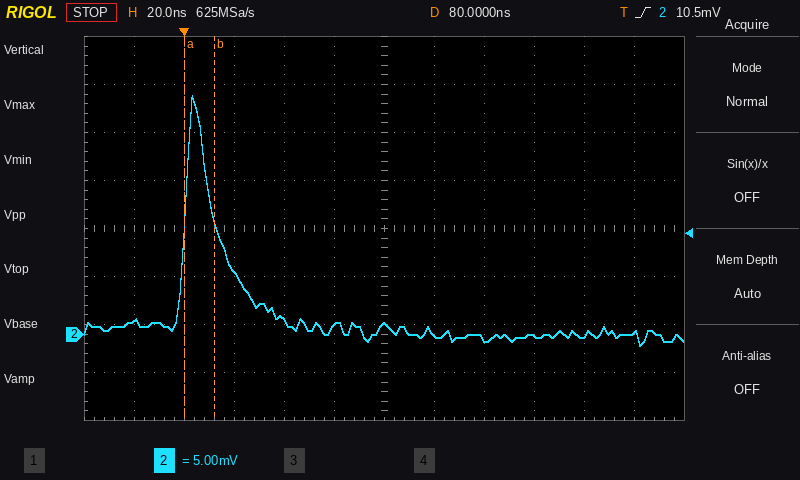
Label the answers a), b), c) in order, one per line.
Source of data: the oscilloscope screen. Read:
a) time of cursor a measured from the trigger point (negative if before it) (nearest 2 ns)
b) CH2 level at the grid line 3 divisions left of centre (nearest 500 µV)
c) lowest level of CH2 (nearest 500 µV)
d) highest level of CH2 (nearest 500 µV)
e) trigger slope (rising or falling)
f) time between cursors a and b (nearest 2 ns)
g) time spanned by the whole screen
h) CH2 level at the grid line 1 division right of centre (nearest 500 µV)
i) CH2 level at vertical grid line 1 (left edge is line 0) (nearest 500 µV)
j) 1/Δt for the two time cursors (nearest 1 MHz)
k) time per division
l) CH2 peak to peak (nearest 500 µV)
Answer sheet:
a) 0 ns
b) 6.5 mV
c) -1.0 mV
d) 25.0 mV
e) rising
f) 12 ns
g) 240 ns
h) 0.0 mV
i) 1.5 mV
j) 83 MHz
k) 20 ns
l) 26.0 mV
